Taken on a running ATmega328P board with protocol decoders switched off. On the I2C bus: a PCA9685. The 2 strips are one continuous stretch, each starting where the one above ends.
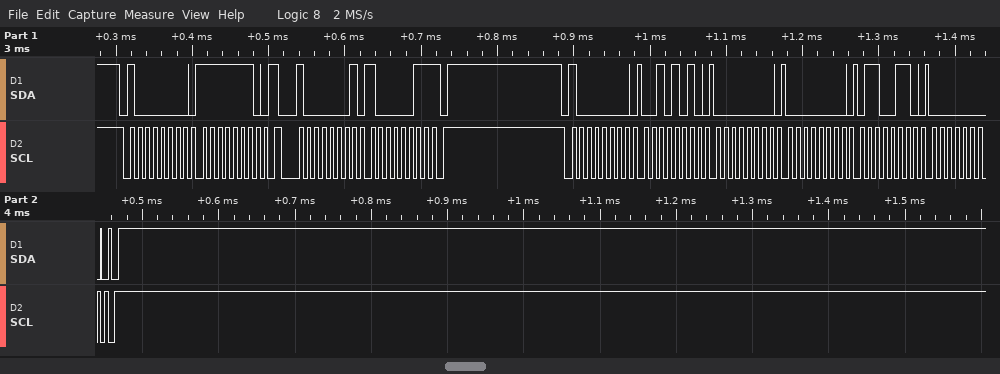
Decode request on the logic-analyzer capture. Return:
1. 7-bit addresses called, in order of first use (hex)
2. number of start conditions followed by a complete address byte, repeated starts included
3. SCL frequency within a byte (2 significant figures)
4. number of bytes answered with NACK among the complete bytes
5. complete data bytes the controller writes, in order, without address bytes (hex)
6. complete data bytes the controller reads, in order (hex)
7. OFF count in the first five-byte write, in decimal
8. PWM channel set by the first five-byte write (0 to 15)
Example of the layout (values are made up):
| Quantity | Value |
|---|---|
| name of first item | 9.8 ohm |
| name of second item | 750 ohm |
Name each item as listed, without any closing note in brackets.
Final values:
| Quantity | Value |
|---|---|
| 7-bit addresses called, in order of first use | 0x40 |
| number of start conditions followed by a complete address byte, repeated starts included | 3 |
| SCL frequency within a byte | 100 kHz |
| number of bytes answered with NACK among the complete bytes | 1 |
| complete data bytes the controller writes, in order, without address bytes | FE 2A 00 00 66 00 |
| complete data bytes the controller reads, in order | 83 |
| OFF count in the first five-byte write, in decimal | 102 |
| PWM channel set by the first five-byte write | 9 |
